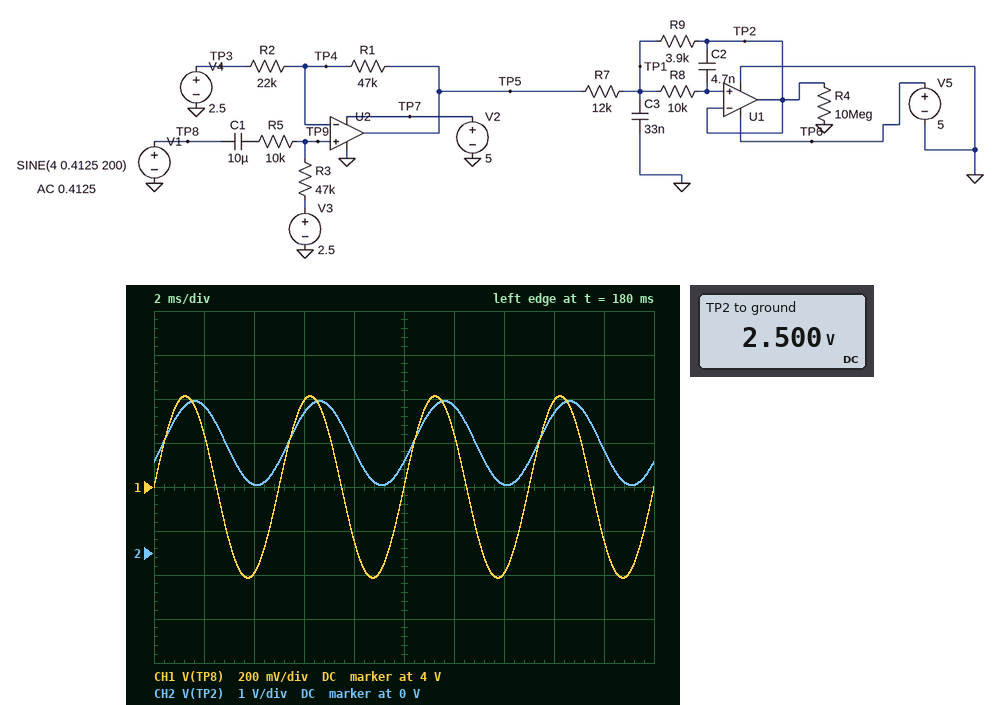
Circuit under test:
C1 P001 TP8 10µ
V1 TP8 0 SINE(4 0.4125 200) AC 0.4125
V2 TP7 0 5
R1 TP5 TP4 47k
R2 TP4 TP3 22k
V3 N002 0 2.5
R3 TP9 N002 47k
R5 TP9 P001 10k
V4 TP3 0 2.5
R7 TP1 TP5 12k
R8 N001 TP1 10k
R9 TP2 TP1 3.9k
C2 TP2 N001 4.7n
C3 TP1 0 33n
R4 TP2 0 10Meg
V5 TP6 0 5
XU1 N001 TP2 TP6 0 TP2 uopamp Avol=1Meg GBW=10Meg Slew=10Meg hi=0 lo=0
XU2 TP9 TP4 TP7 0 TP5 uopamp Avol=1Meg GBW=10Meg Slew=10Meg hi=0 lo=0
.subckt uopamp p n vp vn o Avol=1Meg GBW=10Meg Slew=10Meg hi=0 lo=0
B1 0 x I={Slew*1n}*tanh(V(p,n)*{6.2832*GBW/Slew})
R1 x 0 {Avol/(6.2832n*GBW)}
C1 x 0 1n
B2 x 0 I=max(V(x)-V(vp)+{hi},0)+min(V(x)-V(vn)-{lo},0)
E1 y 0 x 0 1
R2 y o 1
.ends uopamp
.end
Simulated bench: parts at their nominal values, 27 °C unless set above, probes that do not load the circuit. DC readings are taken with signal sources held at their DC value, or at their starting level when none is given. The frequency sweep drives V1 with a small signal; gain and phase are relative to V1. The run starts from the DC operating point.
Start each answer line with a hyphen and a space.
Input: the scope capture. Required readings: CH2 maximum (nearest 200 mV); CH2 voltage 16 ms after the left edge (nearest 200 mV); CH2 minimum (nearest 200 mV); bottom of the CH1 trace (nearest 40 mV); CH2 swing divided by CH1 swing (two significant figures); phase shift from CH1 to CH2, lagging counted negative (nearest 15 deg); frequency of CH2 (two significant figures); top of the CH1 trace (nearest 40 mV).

- 3.4 V
- 3.2 V
- 1.6 V
- 3.60 V
- 2.3
- -30 deg
- 200 Hz
- 4.40 V
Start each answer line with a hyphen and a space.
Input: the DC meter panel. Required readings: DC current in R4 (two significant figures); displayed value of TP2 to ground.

- 250 nA
- 2.500 V
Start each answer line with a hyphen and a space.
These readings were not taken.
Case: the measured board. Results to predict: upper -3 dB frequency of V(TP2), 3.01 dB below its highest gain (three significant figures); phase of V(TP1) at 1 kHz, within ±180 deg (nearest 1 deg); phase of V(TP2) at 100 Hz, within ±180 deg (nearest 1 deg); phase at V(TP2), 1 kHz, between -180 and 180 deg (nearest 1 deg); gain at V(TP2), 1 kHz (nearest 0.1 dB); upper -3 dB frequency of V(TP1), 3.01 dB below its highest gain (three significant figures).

- 402 Hz
- -68 deg
- -14 deg
- -68 deg
- -0.3 dB
- 402 Hz
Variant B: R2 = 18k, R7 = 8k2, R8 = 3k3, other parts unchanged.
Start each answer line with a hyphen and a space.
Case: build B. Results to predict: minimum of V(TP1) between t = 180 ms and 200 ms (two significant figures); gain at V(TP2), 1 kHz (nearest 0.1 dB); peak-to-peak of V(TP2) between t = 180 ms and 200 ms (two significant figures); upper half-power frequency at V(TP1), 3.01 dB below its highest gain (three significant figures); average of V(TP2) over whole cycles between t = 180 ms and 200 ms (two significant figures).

- 1.3 V
- 3.6 dB
- 2.3 V
- 589 Hz
- 2.5 V
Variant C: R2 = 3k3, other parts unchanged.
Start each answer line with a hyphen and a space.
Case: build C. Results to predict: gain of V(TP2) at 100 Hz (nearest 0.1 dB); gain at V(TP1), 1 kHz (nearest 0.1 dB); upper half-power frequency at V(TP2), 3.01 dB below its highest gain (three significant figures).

- 21.7 dB
- 13.4 dB
- 402 Hz
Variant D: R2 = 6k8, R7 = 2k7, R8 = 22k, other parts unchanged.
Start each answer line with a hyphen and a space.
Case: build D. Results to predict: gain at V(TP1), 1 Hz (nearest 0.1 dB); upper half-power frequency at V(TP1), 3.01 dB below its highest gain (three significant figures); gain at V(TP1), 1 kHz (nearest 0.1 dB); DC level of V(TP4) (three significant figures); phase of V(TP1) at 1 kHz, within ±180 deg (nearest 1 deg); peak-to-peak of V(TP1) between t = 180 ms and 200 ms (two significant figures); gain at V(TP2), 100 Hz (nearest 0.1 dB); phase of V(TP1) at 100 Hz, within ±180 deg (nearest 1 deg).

- 16.0 dB
- 1.79 kHz
- 15.1 dB
- 2.50 V
- -29 deg
- 5.0 V
- 16.3 dB
- -3 deg
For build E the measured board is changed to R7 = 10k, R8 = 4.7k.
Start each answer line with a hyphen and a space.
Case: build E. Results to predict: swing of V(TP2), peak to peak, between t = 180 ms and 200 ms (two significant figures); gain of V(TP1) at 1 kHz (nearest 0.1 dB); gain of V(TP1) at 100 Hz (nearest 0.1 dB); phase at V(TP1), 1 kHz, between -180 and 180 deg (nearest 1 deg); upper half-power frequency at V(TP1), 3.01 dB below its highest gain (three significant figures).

- 2.0 V
- 1.0 dB
- 8.1 dB
- -64 deg
- 483 Hz
